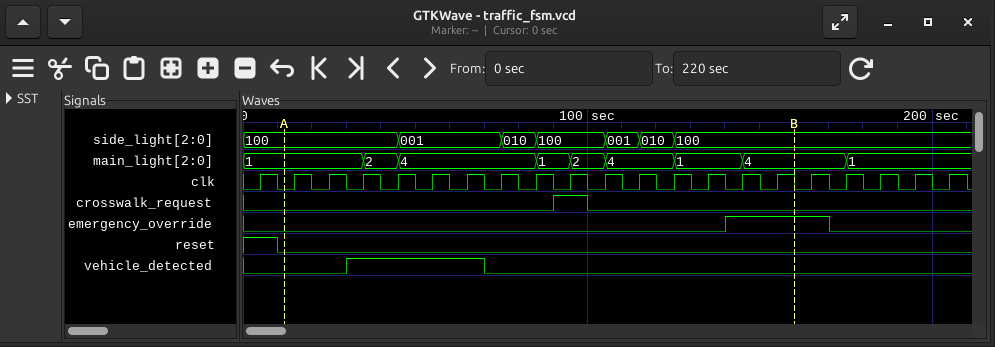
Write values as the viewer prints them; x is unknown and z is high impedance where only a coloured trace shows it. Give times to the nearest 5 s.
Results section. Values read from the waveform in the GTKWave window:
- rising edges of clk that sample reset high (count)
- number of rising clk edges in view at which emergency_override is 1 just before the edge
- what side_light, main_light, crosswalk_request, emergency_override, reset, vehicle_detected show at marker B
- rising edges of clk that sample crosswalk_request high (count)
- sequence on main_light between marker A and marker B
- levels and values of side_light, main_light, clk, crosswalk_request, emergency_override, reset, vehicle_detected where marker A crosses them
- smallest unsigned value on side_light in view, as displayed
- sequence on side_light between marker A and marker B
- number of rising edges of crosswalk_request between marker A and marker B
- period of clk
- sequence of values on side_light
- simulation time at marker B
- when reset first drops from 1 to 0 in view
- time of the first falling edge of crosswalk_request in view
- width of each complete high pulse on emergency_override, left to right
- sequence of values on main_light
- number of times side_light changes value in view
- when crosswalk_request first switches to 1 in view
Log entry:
1
3
side_light=100, main_light=4, crosswalk_request=0, emergency_override=1, reset=0, vehicle_detected=0
1
1, 2, 4, 1, 2, 4, 1, 4
side_light=100, main_light=1, clk=0, crosswalk_request=0, emergency_override=0, reset=0, vehicle_detected=0
001
100, 001, 010, 100, 001, 010, 100
1
10 s
100, 001, 010, 100, 001, 010, 100
160 s
10 s
100 s
30 s
1, 2, 4, 1, 2, 4, 1, 4, 1
6
90 s
